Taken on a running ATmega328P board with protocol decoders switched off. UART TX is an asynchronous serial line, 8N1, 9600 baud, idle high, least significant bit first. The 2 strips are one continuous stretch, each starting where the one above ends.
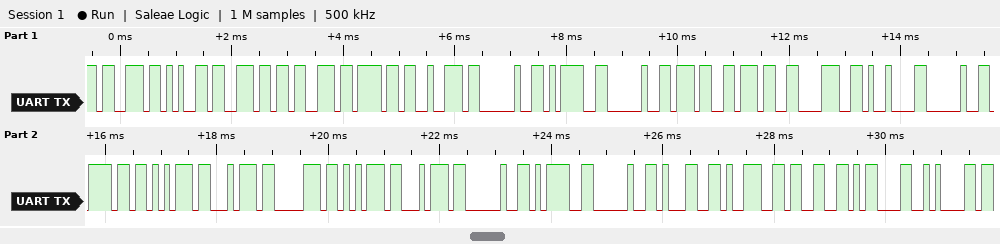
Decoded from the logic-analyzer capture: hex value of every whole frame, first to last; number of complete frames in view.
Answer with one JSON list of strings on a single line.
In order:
["73 65 6E 73 6F 72 20 3D 20 37 37 38 09 20 6F 75 74 70 75 74 20 3D 20 31 39 33 0D 0A", "28"]
